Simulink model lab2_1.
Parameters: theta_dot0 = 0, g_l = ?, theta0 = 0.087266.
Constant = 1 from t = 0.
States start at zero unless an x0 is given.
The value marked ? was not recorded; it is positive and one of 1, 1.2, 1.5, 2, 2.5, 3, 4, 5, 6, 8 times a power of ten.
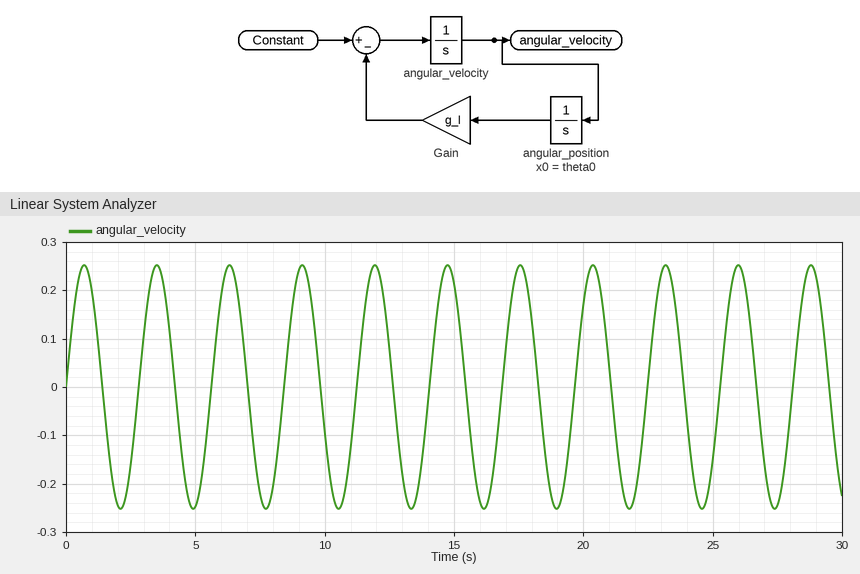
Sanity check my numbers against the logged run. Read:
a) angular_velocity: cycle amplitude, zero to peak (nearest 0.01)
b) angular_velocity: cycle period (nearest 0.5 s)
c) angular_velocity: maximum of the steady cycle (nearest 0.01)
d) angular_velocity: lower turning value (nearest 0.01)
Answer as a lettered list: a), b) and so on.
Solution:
a) 0.25
b) 3.0 s
c) 0.25
d) -0.25
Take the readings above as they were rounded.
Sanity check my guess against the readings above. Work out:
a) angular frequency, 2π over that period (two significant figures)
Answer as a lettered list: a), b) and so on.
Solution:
a) 2.1 rad/s
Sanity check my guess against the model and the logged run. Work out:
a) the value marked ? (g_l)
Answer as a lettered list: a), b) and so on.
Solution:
a) 5
